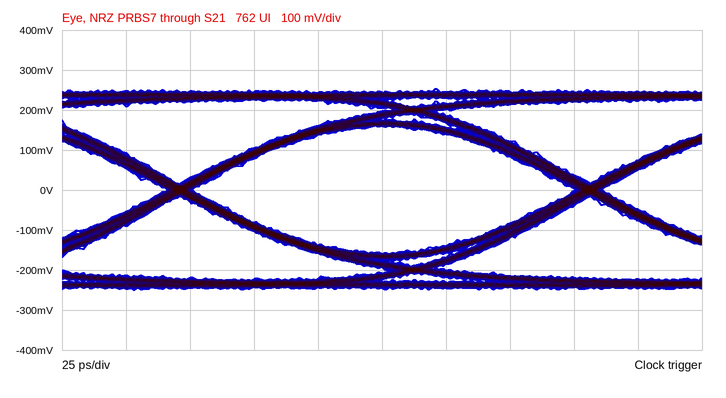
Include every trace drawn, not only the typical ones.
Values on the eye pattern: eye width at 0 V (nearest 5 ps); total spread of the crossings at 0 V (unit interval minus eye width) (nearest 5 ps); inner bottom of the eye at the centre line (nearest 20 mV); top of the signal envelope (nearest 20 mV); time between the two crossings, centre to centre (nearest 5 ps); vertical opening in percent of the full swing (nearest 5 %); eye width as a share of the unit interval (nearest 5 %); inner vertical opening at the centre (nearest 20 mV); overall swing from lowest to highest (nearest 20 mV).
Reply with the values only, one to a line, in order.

150 ps
10 ps
-160 mV
260 mV
160 ps
65 %
95 %
320 mV
500 mV
